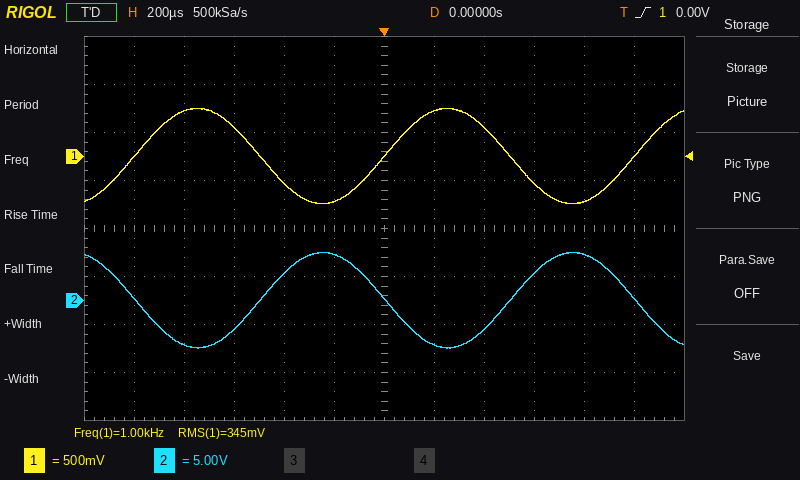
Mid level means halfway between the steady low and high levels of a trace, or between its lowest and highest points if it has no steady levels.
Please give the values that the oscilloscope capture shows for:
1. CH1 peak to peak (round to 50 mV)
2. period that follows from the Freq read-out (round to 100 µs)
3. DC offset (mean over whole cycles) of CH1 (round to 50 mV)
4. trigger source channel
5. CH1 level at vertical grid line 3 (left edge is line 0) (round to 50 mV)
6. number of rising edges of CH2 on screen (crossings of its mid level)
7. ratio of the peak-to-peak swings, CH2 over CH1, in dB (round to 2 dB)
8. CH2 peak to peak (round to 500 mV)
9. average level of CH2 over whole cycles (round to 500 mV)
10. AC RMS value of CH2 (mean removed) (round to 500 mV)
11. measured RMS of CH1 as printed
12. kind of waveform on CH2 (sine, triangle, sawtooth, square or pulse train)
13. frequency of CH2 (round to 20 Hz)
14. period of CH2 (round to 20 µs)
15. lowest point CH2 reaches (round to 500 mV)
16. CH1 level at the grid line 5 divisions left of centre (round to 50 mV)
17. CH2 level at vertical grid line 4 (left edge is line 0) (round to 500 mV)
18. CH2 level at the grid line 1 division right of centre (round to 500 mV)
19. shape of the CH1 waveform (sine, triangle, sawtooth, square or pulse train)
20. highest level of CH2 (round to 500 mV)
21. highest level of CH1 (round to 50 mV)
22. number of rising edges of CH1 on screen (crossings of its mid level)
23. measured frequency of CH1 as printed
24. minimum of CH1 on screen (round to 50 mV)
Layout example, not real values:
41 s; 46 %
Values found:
1.00 V; 1.0 ms; 0 mV; CH1; 300 mV; 2; 20 dB; 10.0 V; 0.0 V; 3.5 V; 345 mV; sine; 1.00 kHz; 1.00 ms; -5.0 V; 0 mV; 3.0 V; -4.5 V; sine; 5.0 V; 500 mV; 3; 1.00 kHz; -500 mV
